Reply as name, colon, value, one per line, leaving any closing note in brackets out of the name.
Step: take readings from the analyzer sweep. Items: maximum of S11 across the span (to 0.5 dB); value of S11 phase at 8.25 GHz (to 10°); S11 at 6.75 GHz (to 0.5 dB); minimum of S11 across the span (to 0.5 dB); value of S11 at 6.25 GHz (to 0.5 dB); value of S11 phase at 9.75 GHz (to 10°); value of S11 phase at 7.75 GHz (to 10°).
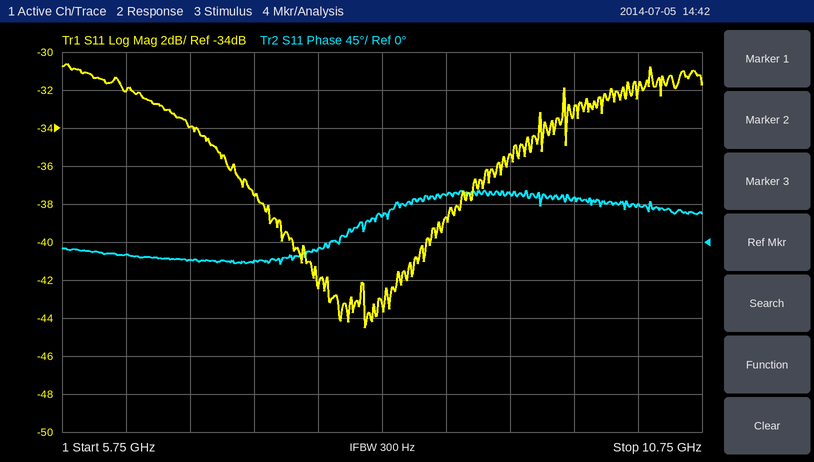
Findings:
maximum of S11 across the span: -30.5 dB
value of S11 phase at 8.25 GHz: 30°
S11 at 6.75 GHz: -34.0 dB
minimum of S11 across the span: -44.5 dB
value of S11 at 6.25 GHz: -32.0 dB
value of S11 phase at 9.75 GHz: 50°
value of S11 phase at 7.75 GHz: -10°
